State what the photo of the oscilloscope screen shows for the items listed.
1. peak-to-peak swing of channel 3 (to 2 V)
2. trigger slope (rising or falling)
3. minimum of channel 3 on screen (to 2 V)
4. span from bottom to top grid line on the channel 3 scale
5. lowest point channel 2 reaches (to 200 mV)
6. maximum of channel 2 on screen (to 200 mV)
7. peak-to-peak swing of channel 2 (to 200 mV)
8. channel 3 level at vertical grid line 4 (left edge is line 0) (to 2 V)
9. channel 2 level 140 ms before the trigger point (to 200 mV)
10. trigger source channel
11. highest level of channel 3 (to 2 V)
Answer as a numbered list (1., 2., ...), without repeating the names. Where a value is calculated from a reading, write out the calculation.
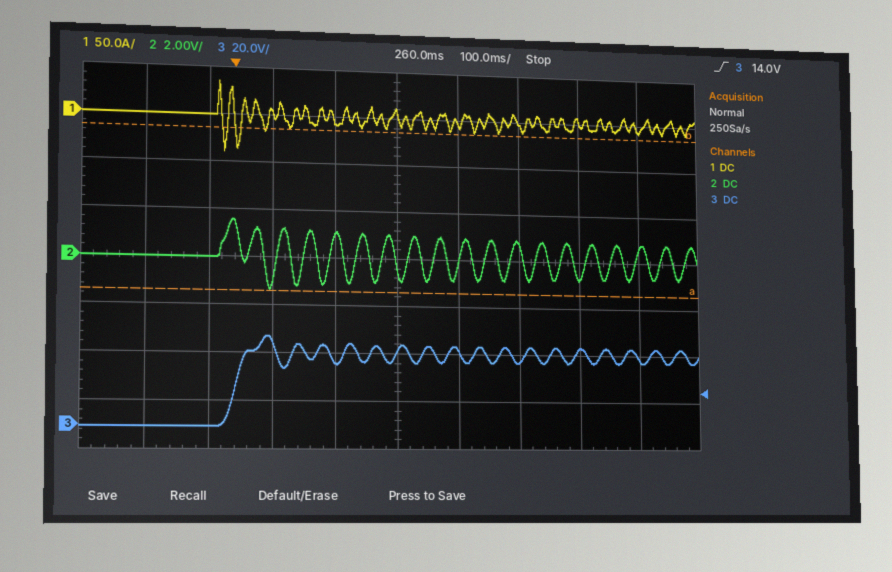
1. 38 V − (0 V) = 38 V
2. rising
3. 0 V
4. 160 V
5. -1.4 V
6. 1.6 V
7. 1.6 V − (-1.4 V) = 3.0 V
8. 26 V
9. 0.0 V
10. channel 3
11. 38 V
